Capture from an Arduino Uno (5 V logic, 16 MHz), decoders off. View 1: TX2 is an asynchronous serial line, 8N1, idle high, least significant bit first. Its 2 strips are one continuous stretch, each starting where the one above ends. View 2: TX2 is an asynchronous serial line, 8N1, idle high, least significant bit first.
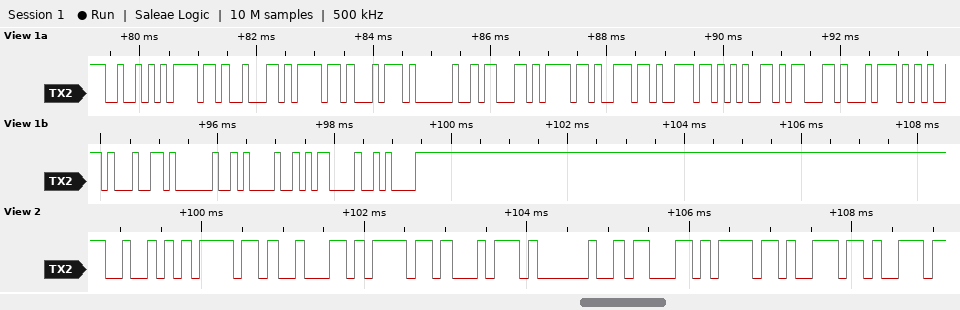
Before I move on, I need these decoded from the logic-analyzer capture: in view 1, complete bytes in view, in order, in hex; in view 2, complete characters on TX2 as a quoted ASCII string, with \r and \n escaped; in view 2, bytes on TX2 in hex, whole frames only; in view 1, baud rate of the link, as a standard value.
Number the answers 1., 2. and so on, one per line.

1. 52 6F 62 6F 74 20 63 6F 6E 6E 65 63 74 65 64 20 21 0D 0A
2. "Robot con"
3. 52 6F 62 6F 74 20 63 6F 6E
4. 9600 baud
